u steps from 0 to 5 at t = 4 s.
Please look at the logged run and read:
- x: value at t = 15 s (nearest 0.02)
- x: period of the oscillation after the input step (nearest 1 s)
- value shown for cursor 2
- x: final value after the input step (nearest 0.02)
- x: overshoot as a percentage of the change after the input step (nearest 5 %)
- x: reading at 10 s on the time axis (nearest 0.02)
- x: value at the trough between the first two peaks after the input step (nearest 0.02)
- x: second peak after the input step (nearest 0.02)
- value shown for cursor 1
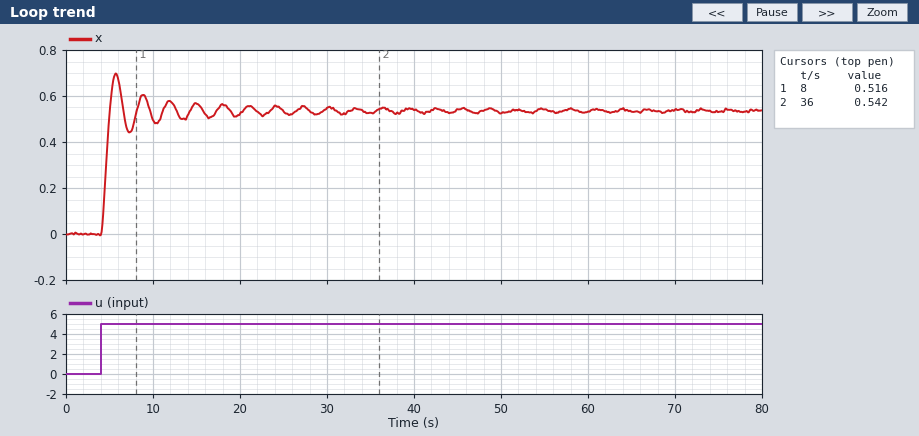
0.56
3 s
0.542
0.54
30 %
0.50
0.44
0.60
0.516
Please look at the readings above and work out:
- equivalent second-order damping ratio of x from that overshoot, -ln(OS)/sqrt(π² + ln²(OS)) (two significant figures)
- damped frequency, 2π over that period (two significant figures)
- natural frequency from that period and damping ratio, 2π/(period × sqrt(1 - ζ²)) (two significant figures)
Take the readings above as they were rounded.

0.36
2.1 rad/s
2.2 rad/s
